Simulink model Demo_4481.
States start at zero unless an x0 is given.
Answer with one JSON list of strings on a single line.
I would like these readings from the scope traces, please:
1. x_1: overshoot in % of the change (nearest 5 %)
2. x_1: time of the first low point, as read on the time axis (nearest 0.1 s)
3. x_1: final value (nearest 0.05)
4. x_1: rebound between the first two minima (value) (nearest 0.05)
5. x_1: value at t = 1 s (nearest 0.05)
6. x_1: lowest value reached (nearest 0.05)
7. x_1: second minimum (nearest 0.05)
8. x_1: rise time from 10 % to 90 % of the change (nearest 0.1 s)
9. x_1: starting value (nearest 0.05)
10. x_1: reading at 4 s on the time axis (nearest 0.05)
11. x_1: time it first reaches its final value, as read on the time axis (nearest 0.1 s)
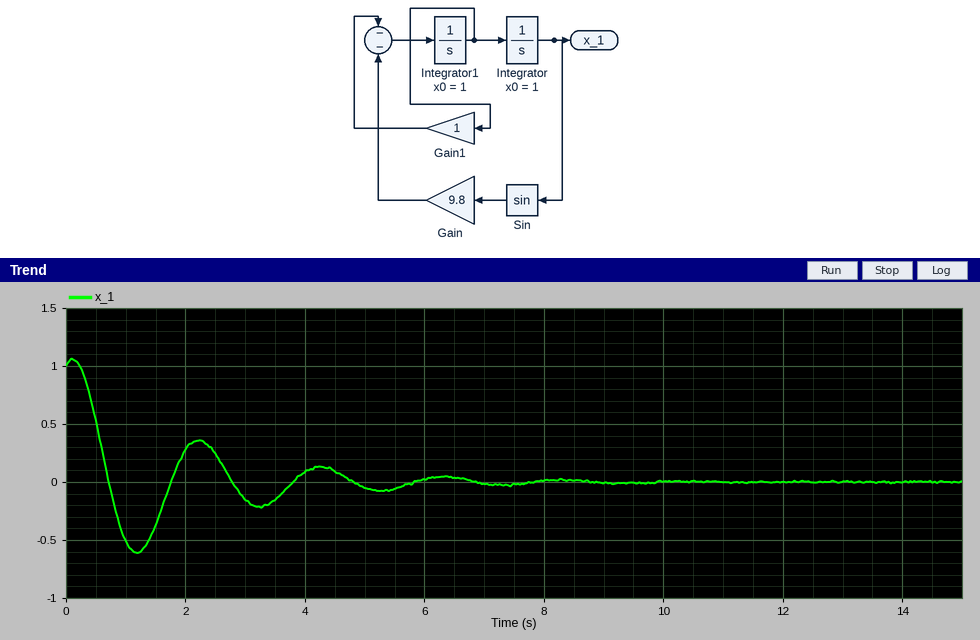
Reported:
["60 %", "1.2 s", "0.00", "0.35", "-0.50", "-0.60", "-0.20", "0.4 s", "1.00", "0.10", "0.7 s"]
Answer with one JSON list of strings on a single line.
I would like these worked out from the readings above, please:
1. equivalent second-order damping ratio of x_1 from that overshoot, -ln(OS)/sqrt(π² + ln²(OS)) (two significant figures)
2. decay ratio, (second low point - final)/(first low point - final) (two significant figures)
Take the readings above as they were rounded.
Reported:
["0.16", "0.33"]
